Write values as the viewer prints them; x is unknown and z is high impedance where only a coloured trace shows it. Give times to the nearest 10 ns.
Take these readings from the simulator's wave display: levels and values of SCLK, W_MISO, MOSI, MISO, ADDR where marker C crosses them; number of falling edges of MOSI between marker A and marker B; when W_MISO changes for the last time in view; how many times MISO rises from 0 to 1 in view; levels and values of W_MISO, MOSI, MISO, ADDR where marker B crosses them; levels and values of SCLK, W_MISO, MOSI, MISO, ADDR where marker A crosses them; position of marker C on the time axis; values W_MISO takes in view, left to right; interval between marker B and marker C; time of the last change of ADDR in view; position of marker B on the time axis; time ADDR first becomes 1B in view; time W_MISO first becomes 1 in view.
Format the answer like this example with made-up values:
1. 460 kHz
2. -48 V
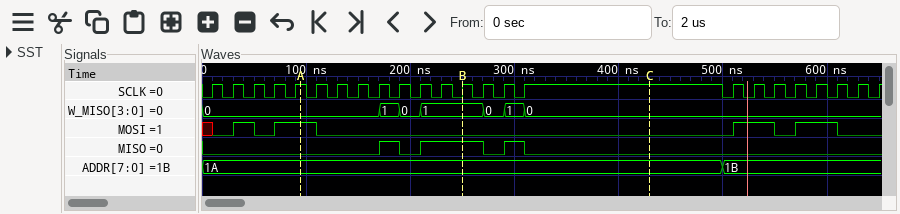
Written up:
1. SCLK=1, W_MISO=0, MOSI=0, MISO=0, ADDR=1A
2. 1
3. 310 ns
4. 3
5. W_MISO=1, MOSI=0, MISO=1, ADDR=1A
6. SCLK=1, W_MISO=0, MOSI=1, MISO=0, ADDR=1A
7. 430 ns
8. 0, 1, 0, 1, 0, 1, 0
9. 180 ns
10. 500 ns
11. 250 ns
12. 500 ns
13. 170 ns
